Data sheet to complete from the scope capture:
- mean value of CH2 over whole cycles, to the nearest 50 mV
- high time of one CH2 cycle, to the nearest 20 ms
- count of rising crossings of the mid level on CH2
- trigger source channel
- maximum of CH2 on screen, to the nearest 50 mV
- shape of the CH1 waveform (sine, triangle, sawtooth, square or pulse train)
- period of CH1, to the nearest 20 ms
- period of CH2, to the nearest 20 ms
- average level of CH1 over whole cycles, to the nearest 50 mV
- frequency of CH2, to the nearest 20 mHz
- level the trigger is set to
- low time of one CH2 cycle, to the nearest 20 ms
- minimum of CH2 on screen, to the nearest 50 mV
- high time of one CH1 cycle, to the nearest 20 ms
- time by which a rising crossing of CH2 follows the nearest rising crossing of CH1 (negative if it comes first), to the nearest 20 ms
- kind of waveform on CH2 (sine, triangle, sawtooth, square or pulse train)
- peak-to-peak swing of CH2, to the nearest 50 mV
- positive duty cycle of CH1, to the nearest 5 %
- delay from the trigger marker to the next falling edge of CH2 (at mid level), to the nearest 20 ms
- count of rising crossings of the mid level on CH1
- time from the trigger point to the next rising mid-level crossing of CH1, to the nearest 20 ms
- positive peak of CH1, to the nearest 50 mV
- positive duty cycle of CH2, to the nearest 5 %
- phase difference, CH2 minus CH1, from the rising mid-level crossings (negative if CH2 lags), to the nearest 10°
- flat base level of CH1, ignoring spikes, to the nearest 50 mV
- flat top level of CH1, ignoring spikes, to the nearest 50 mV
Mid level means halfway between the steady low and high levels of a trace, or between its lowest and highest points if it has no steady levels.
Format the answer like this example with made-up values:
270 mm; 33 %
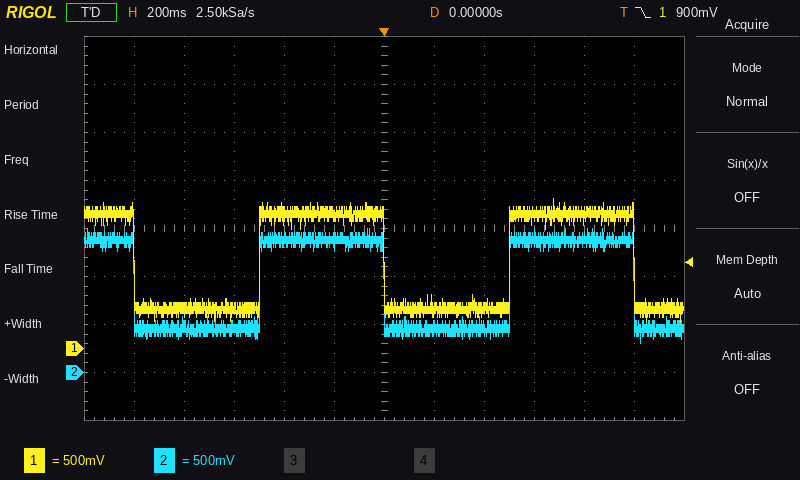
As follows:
900 mV; 500 ms; 2; CH1; 1.50 V; square; 1.00 s; 1.00 s; 900 mV; 1.00 Hz; 900 mV; 500 ms; 300 mV; 500 ms; 0 ms; square; 1.20 V; 50 %; 1.00 s; 2; 500 ms; 1.55 V; 50 %; 0°; 400 mV; 1.40 V
